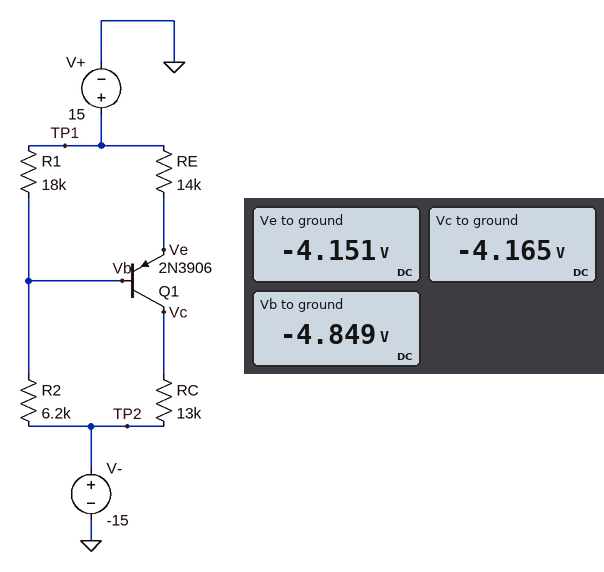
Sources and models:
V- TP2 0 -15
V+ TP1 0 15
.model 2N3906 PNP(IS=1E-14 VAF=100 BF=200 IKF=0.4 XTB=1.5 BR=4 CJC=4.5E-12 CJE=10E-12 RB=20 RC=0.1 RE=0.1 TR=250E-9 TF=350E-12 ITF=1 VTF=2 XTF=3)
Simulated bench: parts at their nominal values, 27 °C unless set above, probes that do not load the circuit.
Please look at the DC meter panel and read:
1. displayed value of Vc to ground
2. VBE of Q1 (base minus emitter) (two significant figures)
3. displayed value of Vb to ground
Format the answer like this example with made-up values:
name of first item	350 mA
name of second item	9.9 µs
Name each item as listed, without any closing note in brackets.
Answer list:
displayed value of Vc to ground	-4.165 V
VBE of Q1 (base minus emitter)	-700 mV
displayed value of Vb to ground	-4.849 V
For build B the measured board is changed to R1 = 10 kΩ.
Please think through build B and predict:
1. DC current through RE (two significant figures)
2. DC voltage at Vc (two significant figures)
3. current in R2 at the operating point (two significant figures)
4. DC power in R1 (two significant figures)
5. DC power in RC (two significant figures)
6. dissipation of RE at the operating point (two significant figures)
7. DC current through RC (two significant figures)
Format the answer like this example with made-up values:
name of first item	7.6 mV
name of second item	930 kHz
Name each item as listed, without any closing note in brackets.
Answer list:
DC current through RE	1.2 mA
DC voltage at Vc	-2.0 V
current in R2 at the operating point	2.0 mA
DC power in R1	31 mW
DC power in RC	13 mW
dissipation of RE at the operating point	21 mW
DC current through RC	1.0 mA
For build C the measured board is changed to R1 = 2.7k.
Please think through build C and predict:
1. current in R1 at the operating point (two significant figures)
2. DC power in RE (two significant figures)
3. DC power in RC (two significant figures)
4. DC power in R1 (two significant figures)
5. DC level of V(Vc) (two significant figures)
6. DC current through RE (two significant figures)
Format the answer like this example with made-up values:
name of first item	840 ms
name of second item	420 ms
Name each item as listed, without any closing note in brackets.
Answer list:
current in R1 at the operating point	3.4 mA
DC power in RE	5.1 mW
DC power in RC	4.7 mW
DC power in R1	31 mW
DC level of V(Vc)	-7.2 V
DC current through RE	600 µA
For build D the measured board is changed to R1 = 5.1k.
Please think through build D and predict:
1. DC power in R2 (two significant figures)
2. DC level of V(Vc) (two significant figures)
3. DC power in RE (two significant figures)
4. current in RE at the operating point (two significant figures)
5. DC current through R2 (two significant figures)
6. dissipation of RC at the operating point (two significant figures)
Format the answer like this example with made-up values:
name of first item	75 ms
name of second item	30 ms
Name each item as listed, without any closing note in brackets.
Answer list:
DC power in R2	44 mW
DC level of V(Vc)	-3.1 V
DC power in RE	12 mW
current in RE at the operating point	920 µA
DC current through R2	2.7 mA
dissipation of RC at the operating point	11 mW
